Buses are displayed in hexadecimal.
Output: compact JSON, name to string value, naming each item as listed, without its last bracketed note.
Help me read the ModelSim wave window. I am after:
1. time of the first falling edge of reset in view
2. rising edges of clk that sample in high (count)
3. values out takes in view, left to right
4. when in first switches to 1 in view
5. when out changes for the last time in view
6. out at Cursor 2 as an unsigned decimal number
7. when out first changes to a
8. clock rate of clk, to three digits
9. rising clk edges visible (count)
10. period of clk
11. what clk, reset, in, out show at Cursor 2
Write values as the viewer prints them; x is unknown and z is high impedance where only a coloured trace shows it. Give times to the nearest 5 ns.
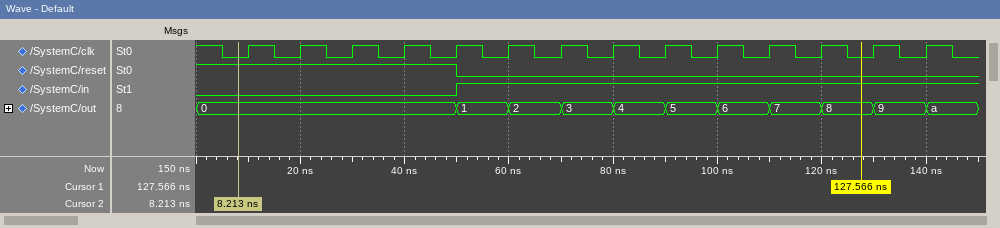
{"time of the first falling edge of reset in view": "50 ns", "rising edges of clk that sample in high": "9", "values out takes in view, left to right": "0, 1, 2, 3, 4, 5, 6, 7, 8, 9, a", "when in first switches to 1 in view": "50 ns", "when out changes for the last time in view": "140 ns", "out at Cursor 2 as an unsigned decimal number": "0", "when out first changes to a": "140 ns", "clock rate of clk, to three digits": "100 MHz", "rising clk edges visible": "14", "period of clk": "10 ns", "what clk, reset, in, out show at Cursor 2": "clk=0, reset=1, in=0, out=0"}
